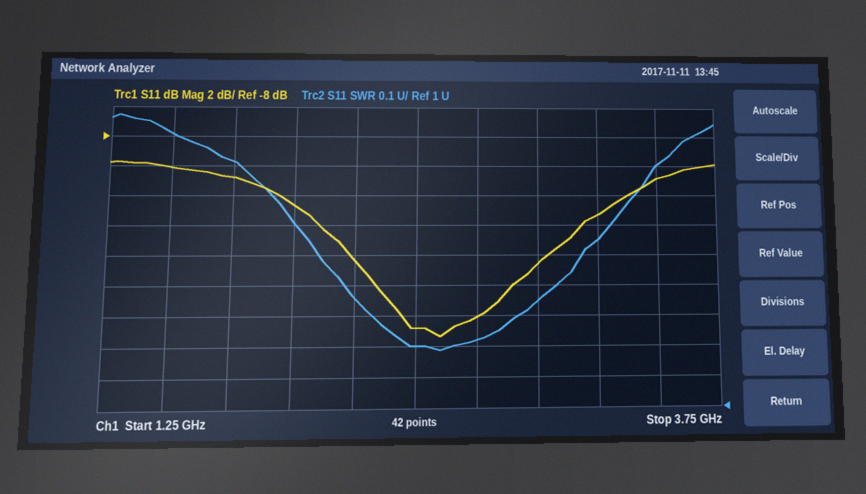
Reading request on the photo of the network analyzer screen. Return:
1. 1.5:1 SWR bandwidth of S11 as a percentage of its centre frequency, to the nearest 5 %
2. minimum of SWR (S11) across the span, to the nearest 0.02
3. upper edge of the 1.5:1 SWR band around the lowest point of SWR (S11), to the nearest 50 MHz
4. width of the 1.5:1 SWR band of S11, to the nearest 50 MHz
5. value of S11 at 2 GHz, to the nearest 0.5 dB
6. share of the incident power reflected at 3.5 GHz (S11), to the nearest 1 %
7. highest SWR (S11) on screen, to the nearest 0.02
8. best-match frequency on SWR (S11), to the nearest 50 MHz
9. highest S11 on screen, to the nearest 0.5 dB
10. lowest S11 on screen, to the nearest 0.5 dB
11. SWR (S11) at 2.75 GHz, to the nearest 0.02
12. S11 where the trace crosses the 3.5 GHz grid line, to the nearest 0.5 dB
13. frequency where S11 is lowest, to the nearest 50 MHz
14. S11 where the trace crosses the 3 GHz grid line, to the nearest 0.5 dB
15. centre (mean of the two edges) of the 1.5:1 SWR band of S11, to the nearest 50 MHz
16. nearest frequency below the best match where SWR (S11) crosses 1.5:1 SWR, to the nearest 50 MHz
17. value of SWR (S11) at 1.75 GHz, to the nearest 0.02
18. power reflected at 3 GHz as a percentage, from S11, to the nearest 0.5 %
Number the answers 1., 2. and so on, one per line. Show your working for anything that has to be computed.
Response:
1. 1.1 GHz / 2.65 GHz ≈ 41.5 %, so 40 % to the nearest 5 %
2. 1.18
3. 3.20 GHz
4. 3.20 GHz − 2.10 GHz = 1.10 GHz
5. -12.5 dB
6. 10^(-11/10) ≈ 8 %
7. 1.98
8. 2.60 GHz
9. -9.5 dB
10. -21.5 dB
11. 1.22
12. -11.0 dB
13. 2.60 GHz
14. -16.5 dB
15. 2.65 GHz
16. 2.10 GHz
17. 1.82
18. 10^(-16.5/10) ≈ 2.24 %, so 2.0 % to the nearest 0.5 %
